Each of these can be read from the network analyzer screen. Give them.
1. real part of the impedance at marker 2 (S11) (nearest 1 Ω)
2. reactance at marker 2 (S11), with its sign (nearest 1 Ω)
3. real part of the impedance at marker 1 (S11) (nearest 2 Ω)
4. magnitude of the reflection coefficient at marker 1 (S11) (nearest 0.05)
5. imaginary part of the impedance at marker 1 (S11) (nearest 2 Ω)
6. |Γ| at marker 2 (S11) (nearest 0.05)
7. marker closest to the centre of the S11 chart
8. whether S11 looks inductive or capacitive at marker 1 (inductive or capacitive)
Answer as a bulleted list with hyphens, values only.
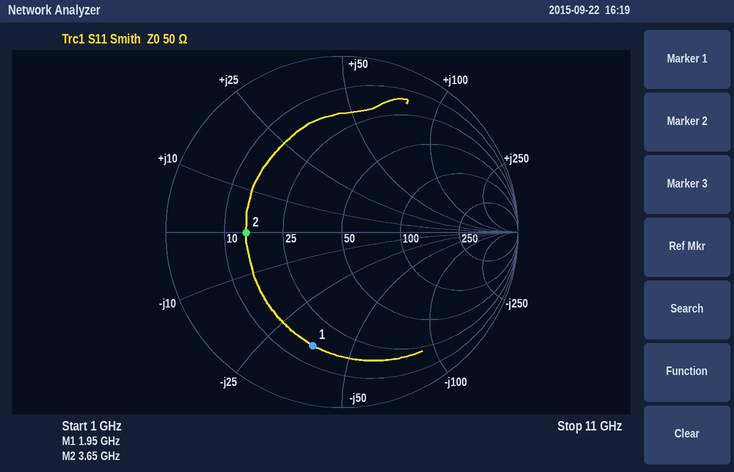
- 15 Ω
- 0 Ω
- 16 Ω
- 0.65
- -36 Ω
- 0.55
- marker 2
- capacitive
